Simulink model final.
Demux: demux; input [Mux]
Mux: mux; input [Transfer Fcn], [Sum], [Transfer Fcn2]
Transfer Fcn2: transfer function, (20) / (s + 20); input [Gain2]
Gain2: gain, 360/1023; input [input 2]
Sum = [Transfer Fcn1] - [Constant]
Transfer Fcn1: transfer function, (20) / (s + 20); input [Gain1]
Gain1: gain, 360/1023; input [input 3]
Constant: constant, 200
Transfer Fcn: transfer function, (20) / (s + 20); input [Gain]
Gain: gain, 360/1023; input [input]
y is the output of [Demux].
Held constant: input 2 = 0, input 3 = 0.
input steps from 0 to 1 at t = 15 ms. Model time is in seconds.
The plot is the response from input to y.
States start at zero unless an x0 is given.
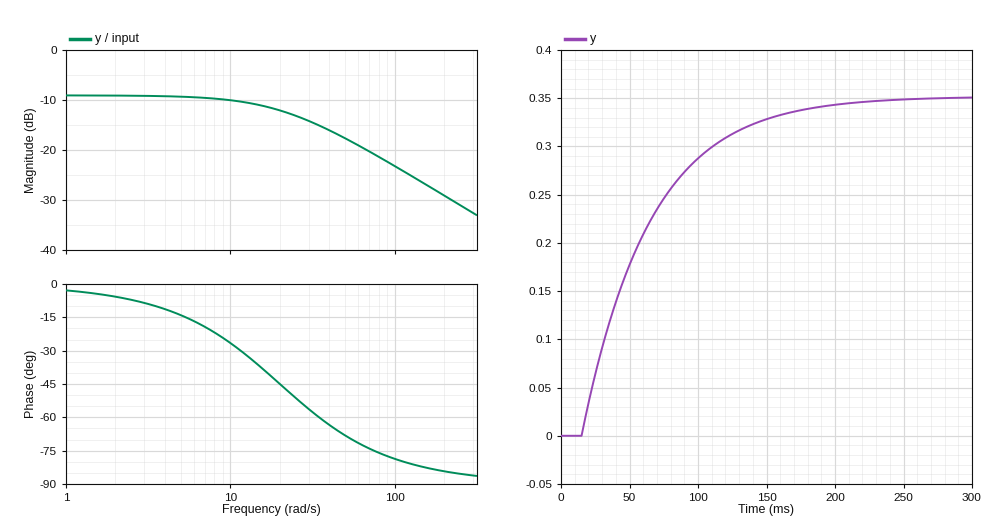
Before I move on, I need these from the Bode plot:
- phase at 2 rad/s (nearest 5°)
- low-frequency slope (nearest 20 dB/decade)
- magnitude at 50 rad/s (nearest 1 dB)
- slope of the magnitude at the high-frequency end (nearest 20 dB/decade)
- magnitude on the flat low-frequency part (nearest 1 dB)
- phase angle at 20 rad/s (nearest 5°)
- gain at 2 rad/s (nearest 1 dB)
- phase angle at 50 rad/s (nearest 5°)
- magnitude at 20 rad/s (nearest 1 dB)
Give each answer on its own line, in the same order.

-5°
0 dB/decade
-18 dB
-20 dB/decade
-9 dB
-45°
-9 dB
-70°
-12 dB
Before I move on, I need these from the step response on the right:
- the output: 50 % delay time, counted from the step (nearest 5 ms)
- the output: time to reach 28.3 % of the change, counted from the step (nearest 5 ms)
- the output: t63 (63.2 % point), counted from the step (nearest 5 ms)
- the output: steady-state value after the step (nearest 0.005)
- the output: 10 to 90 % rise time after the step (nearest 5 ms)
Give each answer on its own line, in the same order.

35 ms
15 ms
50 ms
0.350
110 ms
